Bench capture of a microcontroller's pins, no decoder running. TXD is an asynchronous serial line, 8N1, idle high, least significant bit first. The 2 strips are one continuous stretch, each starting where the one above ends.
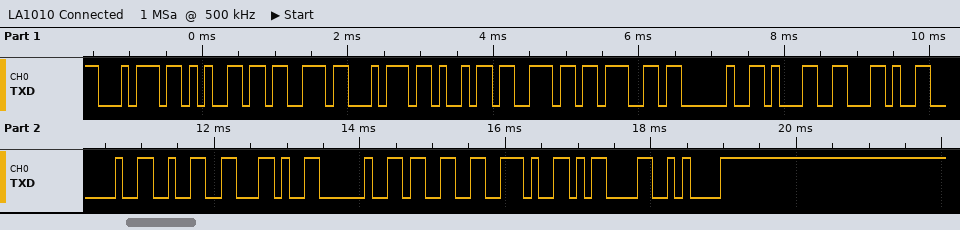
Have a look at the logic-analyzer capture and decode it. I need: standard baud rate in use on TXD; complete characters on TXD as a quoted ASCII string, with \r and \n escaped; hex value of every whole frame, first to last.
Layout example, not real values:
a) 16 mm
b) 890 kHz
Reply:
a) 9600 baud
b) "testing 1, 2, 3.\r\n"
c) 74 65 73 74 69 6E 67 20 31 2C 20 32 2C 20 33 2E 0D 0A
